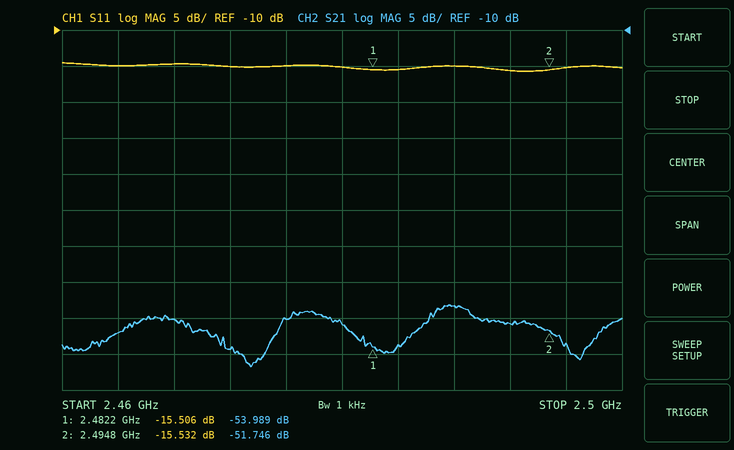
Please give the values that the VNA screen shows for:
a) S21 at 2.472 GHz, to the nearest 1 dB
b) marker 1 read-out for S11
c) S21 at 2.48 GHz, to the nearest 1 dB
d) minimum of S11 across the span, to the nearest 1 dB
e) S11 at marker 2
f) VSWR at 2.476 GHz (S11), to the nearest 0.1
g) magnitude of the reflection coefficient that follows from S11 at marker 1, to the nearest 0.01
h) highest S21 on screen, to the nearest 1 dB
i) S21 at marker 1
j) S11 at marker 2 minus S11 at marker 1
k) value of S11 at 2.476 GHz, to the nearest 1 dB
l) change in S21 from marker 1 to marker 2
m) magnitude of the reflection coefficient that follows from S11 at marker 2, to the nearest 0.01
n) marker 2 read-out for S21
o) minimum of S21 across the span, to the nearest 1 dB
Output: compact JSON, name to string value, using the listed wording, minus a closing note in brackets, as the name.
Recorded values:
{"S21 at 2.472 GHz, to the nearest 1 dB": "-54 dB", "marker 1 read-out for S11": "-15.506 dB", "S21 at 2.48 GHz, to the nearest 1 dB": "-51 dB", "minimum of S11 across the span, to the nearest 1 dB": "-16 dB", "S11 at marker 2": "-15.532 dB", "VSWR at 2.476 GHz (S11), to the nearest 0.1": "1.4", "magnitude of the reflection coefficient that follows from S11 at marker 1, to the nearest 0.01": "0.17", "highest S21 on screen, to the nearest 1 dB": "-48 dB", "S21 at marker 1": "-53.989 dB", "S11 at marker 2 minus S11 at marker 1": "-0.026 dB", "value of S11 at 2.476 GHz, to the nearest 1 dB": "-15 dB", "change in S21 from marker 1 to marker 2": "2.243 dB", "magnitude of the reflection coefficient that follows from S11 at marker 2, to the nearest 0.01": "0.17", "marker 2 read-out for S21": "-51.746 dB", "minimum of S21 across the span, to the nearest 1 dB": "-57 dB"}
